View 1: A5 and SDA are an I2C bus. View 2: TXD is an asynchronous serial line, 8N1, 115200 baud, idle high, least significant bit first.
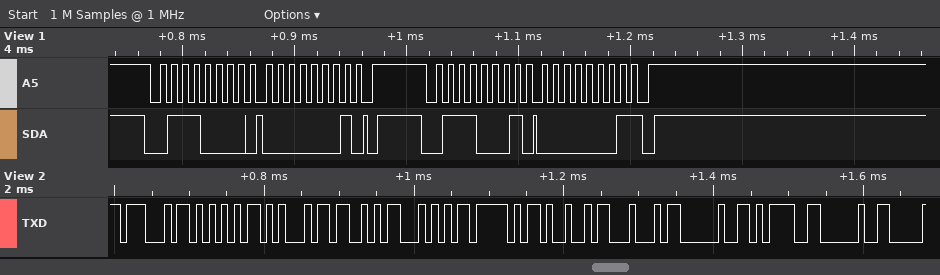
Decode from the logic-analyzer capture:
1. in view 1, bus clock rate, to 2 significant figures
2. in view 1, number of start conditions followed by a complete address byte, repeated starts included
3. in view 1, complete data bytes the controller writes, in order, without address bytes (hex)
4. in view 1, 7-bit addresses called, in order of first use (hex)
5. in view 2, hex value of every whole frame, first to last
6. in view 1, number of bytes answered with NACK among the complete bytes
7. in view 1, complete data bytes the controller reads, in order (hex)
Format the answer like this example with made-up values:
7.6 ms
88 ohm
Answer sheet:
100 kHz
2
01
0x38
47 55 45 53 54 5F 49 44 20 3D 20
1
01
